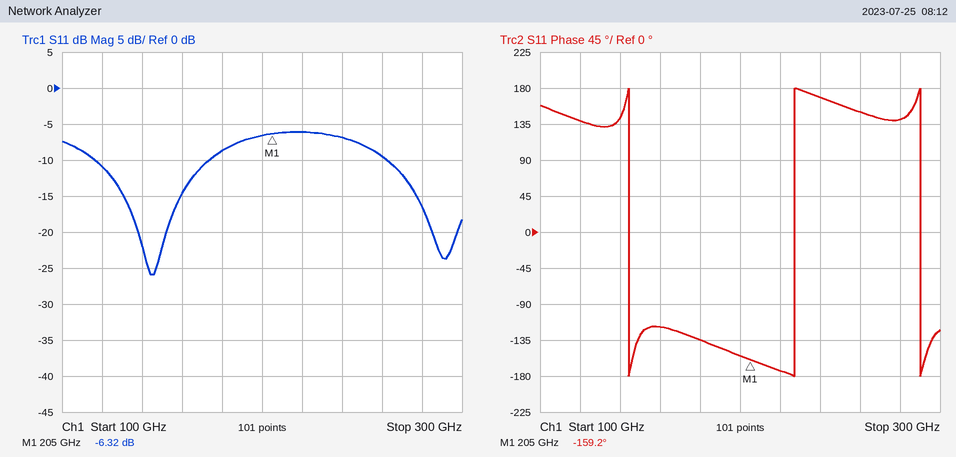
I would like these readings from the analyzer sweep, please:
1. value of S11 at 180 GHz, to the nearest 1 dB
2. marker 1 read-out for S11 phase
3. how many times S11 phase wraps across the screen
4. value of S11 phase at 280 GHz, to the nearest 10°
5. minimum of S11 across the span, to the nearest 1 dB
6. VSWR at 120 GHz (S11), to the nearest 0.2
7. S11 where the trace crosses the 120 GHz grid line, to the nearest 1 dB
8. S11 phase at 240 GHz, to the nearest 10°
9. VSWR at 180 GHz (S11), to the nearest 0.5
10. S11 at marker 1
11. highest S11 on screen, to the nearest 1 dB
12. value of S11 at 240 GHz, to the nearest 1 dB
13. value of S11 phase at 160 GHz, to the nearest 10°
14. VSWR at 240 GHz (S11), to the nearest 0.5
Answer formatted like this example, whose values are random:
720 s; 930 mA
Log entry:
-9 dB; -159.2°; 3; 140°; -26 dB; 1.8; -11 dB; 170°; 2.0; -6.32 dB; -6 dB; -7 dB; -120°; 2.5
